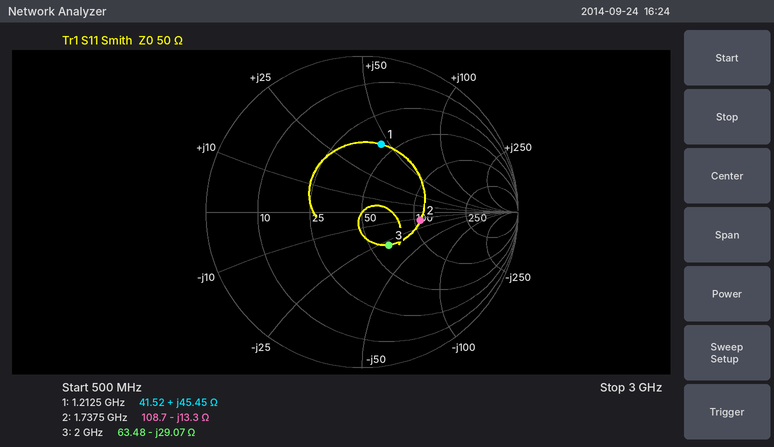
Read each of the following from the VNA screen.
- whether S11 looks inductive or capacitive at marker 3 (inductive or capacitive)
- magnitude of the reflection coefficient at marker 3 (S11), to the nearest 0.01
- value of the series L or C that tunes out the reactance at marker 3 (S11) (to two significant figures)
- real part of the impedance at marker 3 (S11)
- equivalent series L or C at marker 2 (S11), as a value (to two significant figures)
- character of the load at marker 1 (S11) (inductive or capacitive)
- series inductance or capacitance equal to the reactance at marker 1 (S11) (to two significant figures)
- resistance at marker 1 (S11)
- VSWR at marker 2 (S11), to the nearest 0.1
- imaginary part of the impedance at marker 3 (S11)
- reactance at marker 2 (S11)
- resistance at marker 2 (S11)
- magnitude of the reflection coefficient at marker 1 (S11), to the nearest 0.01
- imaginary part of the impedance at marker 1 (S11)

capacitive
0.27
2.3 nH
63.48 Ω
6.9 pF
inductive
6.0 nH
41.52 Ω
2.2
-29.07 Ω
-13.3 Ω
108.7 Ω
0.45
+45.45 Ω
